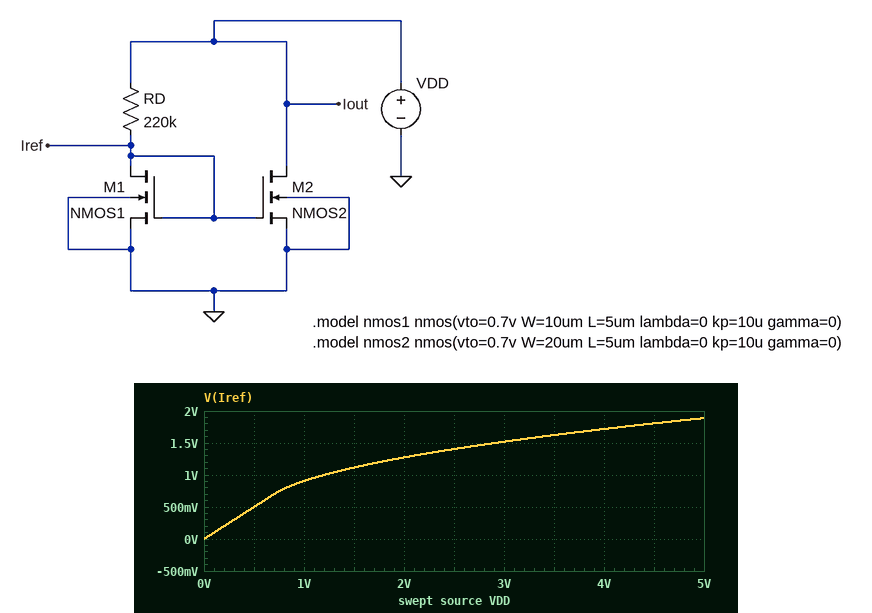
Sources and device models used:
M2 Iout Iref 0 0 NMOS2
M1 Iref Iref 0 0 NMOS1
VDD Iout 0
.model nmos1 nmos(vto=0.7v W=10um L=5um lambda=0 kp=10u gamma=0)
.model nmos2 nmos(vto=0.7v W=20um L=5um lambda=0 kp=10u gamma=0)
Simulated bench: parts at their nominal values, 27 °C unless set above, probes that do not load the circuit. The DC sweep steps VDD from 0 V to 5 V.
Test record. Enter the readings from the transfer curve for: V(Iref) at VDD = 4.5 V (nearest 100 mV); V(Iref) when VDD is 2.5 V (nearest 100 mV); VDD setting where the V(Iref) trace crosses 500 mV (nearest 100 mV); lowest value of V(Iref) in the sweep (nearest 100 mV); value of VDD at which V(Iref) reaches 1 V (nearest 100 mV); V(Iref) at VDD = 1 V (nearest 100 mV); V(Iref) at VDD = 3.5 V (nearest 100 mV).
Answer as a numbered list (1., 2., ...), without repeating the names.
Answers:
1. 1.8 V
2. 1.4 V
3. 500 mV
4. 0 V
5. 1.2 V
6. 900 mV
7. 1.6 V
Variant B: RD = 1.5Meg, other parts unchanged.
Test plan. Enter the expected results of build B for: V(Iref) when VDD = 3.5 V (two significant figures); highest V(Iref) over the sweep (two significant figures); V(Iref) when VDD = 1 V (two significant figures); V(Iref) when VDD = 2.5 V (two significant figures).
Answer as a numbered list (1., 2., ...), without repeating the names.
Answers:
1. 1.1 V
2. 1.2 V
3. 810 mV
4. 1.0 V
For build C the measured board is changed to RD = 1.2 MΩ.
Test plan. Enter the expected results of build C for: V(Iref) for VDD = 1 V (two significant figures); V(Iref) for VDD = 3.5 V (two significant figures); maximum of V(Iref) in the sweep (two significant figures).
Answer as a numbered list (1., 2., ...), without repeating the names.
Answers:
1. 820 mV
2. 1.1 V
3. 1.3 V
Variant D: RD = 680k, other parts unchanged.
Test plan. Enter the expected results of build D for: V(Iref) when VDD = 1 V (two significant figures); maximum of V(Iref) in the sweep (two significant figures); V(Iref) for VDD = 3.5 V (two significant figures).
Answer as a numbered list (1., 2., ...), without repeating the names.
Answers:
1. 850 mV
2. 1.4 V
3. 1.3 V
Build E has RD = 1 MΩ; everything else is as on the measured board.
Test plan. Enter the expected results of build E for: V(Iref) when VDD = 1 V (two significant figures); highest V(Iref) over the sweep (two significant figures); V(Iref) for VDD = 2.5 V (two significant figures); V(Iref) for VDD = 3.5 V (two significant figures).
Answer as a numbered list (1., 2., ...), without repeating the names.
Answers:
1. 830 mV
2. 1.3 V
3. 1.1 V
4. 1.2 V
